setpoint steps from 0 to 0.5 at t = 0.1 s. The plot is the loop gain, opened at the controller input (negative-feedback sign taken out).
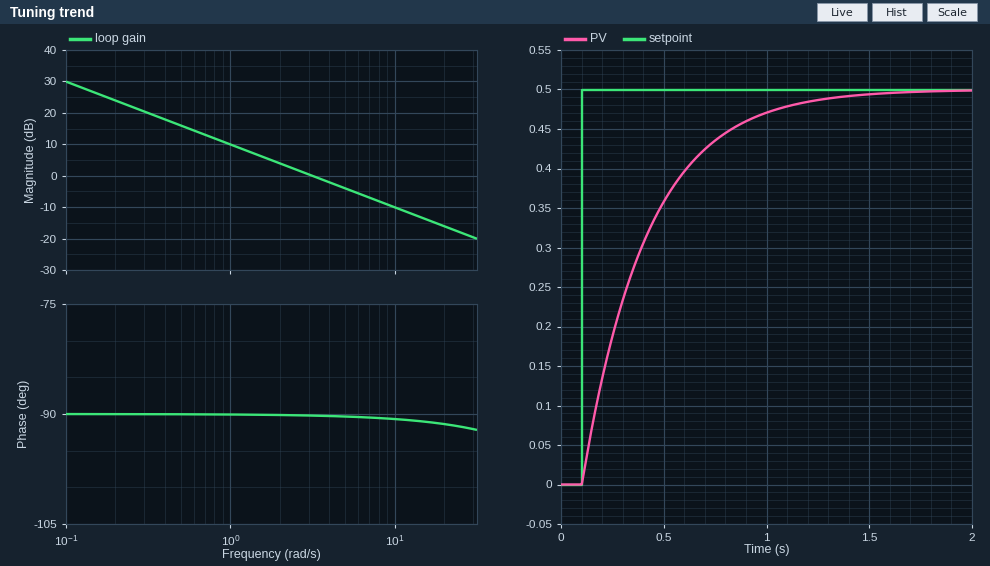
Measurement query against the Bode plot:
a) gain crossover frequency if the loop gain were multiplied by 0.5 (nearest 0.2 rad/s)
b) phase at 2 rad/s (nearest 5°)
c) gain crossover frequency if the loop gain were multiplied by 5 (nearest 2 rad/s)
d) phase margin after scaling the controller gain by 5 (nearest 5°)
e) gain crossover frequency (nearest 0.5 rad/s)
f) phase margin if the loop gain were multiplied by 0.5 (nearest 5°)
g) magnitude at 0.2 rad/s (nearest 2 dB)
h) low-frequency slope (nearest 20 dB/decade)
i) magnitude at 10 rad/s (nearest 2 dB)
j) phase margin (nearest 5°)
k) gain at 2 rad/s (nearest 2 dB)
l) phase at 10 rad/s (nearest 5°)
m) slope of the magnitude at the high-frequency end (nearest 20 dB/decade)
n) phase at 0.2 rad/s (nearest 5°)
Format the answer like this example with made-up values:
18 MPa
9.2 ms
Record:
1.6 rad/s
-90°
16 rad/s
90°
3.0 rad/s
90°
24 dB
-20 dB/decade
-10 dB
90°
4 dB
-90°
-20 dB/decade
-90°
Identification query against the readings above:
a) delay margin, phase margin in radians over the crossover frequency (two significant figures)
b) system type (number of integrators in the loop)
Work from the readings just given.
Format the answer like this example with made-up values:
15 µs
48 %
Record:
0.52 s
1
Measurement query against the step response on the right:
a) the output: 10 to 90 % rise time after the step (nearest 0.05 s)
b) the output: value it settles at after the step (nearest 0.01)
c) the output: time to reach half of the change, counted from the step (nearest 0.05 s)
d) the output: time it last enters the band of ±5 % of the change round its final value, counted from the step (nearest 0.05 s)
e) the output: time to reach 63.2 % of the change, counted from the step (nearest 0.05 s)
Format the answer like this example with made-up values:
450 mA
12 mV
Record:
0.70 s
0.50
0.20 s
0.95 s
0.30 s
